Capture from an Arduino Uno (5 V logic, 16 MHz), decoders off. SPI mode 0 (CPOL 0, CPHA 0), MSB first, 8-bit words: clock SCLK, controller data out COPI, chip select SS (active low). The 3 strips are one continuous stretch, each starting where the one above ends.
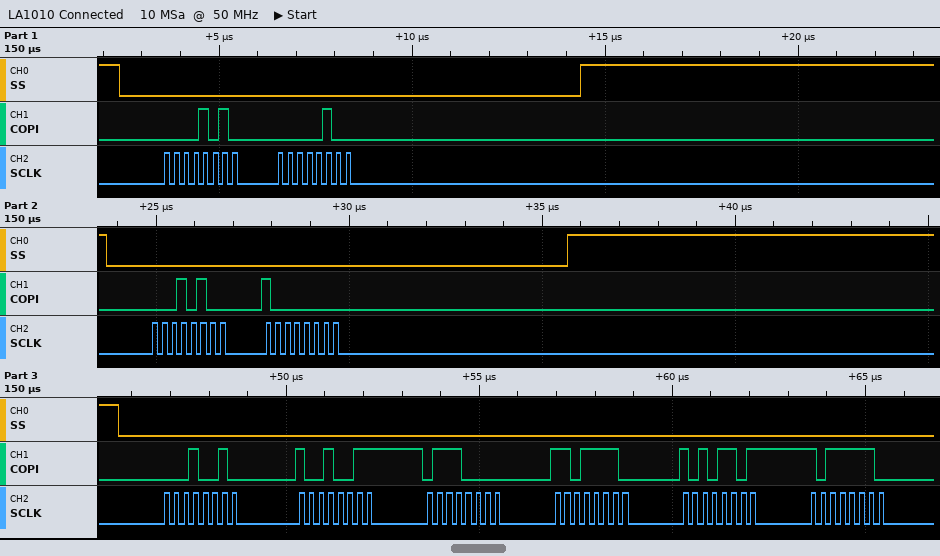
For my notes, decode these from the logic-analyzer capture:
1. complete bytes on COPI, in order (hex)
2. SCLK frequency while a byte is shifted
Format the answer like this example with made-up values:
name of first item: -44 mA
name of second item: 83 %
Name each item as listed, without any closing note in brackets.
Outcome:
complete bytes on COPI, in order: 0A 04 14 80 12 93 70 DE AD BE
SCLK frequency while a byte is shifted: 4 MHz
